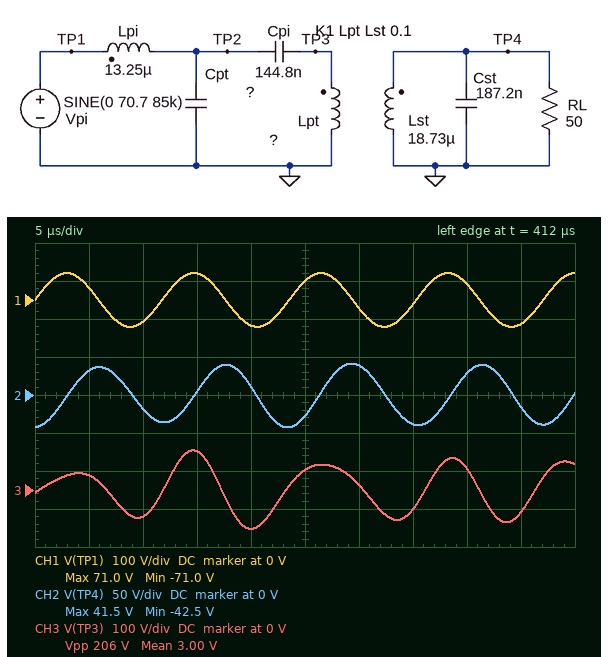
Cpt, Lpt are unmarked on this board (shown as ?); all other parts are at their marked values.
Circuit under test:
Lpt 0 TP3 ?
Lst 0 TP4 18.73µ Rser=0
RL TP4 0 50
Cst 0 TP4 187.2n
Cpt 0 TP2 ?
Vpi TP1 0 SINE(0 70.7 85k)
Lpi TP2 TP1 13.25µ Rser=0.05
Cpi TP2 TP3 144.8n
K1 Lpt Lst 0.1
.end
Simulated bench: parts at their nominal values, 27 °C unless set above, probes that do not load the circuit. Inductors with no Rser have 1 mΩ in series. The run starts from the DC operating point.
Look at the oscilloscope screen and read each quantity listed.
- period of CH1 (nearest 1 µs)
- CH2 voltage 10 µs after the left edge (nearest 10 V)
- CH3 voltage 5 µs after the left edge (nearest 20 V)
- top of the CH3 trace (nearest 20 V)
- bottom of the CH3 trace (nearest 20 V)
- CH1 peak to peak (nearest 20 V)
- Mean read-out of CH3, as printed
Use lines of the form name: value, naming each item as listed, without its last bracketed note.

period of CH1: 12 µs
CH2 voltage 10 µs after the left edge: -20 V
CH3 voltage 5 µs after the left edge: 40 V
top of the CH3 trace: 100 V
bottom of the CH3 trace: -100 V
CH1 peak to peak: 140 V
Mean read-out of CH3, as printed: 3.00 V
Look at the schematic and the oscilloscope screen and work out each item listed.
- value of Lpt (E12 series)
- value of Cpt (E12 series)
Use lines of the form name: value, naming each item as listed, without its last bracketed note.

value of Lpt: 18 µH
value of Cpt: 390 nF
